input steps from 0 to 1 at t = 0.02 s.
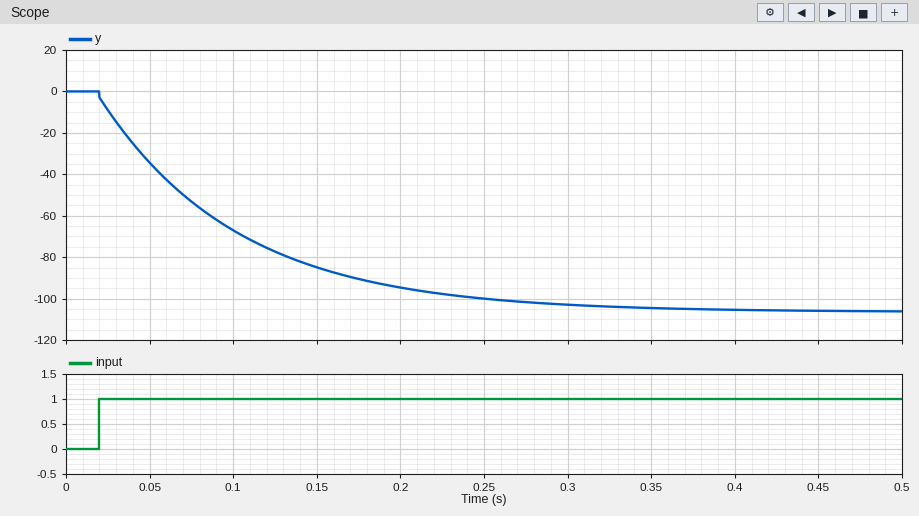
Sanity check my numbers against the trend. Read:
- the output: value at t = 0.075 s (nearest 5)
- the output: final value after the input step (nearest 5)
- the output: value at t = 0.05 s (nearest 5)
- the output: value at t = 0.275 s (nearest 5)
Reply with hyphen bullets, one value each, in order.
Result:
- -55
- -105
- -35
- -100
